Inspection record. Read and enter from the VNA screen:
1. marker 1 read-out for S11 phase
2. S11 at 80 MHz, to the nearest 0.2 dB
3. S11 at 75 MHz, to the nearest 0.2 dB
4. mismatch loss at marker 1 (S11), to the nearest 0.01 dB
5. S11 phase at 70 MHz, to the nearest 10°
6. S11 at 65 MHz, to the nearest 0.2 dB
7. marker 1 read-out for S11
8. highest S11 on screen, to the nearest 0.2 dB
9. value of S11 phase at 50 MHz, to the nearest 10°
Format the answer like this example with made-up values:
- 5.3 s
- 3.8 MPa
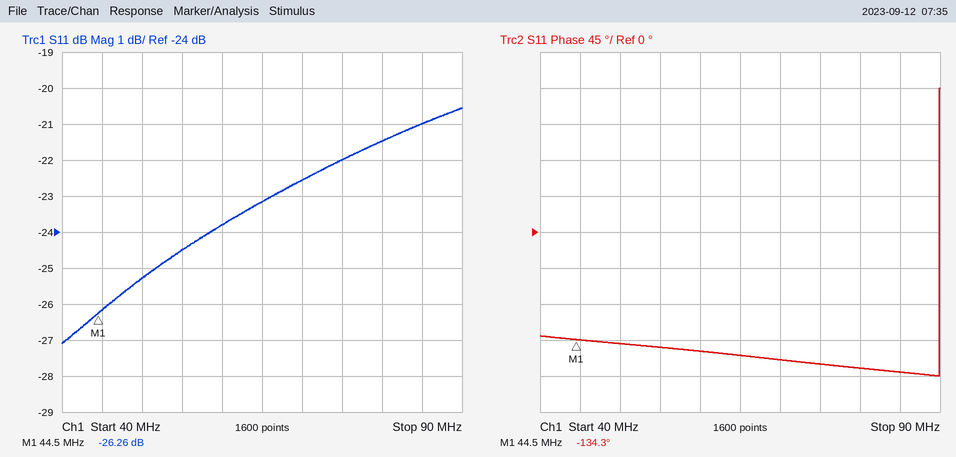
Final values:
- -134.3°
- -21.4 dB
- -22.0 dB
- 0.01 dB
- -160°
- -23.2 dB
- -26.26 dB
- -20.6 dB
- -140°
